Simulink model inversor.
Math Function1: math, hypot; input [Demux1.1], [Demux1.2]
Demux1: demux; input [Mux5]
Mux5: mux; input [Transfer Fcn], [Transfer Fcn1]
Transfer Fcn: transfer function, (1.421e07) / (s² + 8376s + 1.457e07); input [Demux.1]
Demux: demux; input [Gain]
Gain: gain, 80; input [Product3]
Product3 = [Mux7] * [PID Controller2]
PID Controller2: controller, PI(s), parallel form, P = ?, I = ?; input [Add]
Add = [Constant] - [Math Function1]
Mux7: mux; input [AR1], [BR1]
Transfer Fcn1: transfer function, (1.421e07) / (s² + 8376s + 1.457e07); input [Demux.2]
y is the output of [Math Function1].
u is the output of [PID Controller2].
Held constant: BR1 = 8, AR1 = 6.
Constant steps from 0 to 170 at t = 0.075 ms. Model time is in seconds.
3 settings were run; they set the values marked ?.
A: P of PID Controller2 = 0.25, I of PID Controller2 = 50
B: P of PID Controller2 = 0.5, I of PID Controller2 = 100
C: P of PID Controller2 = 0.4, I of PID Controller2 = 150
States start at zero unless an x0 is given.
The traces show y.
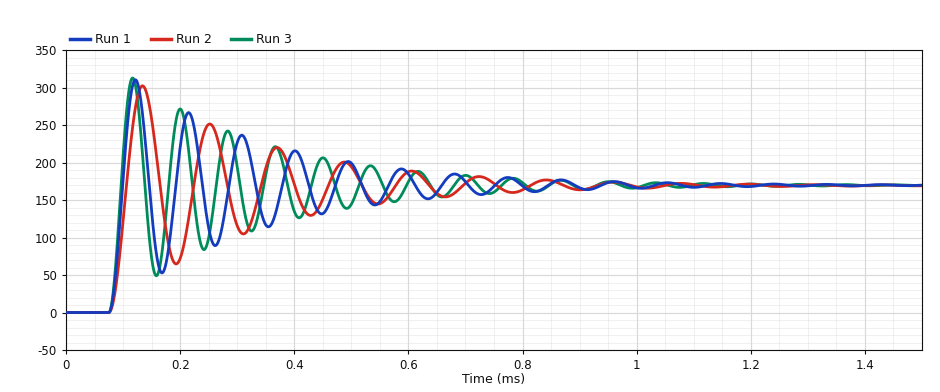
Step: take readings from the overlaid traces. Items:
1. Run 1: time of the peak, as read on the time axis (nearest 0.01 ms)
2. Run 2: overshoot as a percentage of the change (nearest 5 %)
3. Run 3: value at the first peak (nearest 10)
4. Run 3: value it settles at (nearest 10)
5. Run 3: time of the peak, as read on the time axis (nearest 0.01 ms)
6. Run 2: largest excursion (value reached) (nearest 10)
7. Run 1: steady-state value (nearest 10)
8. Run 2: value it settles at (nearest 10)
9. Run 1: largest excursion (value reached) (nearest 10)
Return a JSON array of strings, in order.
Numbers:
["0.12 ms", "80 %", "310", "170", "0.12 ms", "300", "170", "170", "310"]
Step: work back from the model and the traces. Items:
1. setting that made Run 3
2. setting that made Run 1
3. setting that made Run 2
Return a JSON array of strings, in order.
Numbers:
["B", "C", "A"]
